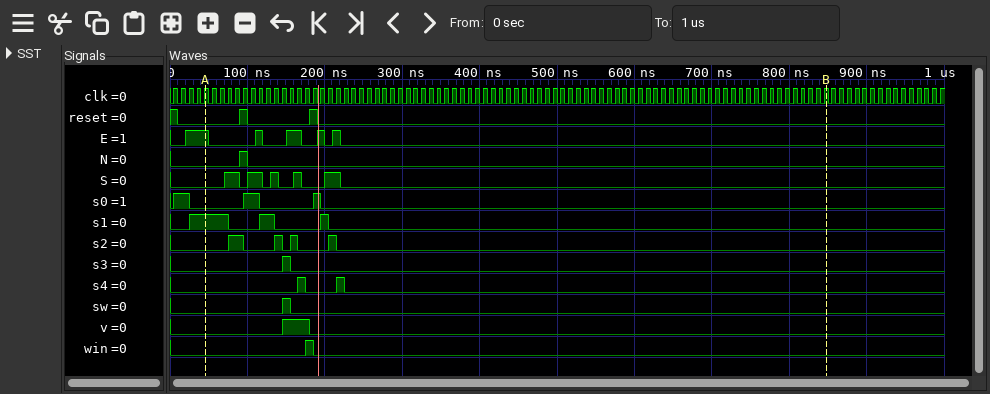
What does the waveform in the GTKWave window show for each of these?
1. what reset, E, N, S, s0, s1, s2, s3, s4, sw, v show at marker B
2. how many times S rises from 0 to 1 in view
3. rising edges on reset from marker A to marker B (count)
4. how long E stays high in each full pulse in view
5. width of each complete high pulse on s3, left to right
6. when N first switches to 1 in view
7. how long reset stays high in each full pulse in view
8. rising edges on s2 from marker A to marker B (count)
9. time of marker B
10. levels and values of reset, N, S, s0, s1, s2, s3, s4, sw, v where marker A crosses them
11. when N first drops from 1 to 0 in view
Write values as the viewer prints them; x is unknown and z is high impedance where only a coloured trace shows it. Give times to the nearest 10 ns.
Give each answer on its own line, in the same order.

reset=0, E=0, N=0, S=0, s0=0, s1=0, s2=0, s3=0, s4=0, sw=0, v=0
5
2
30 ns, 10 ns, 20 ns, 10 ns, 10 ns
10 ns
90 ns
10 ns, 10 ns
4
850 ns
reset=0, N=0, S=0, s0=0, s1=1, s2=0, s3=0, s4=0, sw=0, v=0
100 ns
